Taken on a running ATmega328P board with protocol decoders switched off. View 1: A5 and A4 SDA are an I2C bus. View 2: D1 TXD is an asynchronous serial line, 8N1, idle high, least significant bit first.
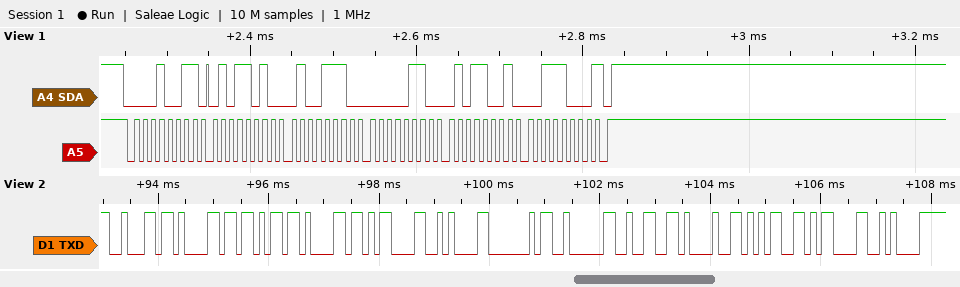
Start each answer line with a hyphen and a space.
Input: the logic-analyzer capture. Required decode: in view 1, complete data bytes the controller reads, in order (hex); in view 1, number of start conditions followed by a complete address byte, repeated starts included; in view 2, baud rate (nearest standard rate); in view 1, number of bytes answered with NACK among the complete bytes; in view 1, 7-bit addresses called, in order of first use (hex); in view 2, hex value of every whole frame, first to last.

- 5A 4E 06 59 38
- 1
- 9600 baud
- 1
- 0x09
- 62 61 6B 61 0D 0A 40 02 32 21 35 0D 0A
